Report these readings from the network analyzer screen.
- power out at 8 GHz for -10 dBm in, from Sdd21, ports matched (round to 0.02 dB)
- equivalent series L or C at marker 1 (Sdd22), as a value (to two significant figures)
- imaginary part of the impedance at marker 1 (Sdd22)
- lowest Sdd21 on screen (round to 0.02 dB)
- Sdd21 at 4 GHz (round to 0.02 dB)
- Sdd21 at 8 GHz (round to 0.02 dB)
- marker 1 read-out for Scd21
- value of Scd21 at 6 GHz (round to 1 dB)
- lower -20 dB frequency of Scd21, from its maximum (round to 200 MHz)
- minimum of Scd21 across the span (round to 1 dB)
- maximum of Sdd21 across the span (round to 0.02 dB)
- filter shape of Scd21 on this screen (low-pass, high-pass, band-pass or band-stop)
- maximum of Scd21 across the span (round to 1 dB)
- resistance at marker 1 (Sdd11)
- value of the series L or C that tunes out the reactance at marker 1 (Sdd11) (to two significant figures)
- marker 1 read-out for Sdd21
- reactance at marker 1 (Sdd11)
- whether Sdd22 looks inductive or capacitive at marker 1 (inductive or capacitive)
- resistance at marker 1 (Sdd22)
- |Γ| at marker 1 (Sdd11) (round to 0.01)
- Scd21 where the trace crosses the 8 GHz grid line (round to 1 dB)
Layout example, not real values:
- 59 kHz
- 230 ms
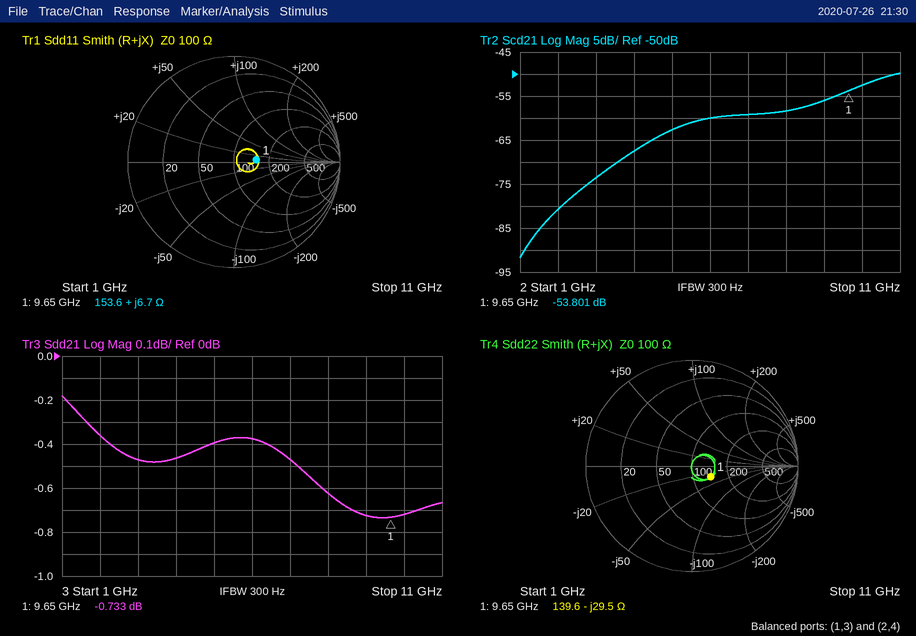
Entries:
- -10.62 dBm
- 560 fF
- -29.5 Ω
- -0.74 dB
- -0.46 dB
- -0.62 dB
- -53.801 dB
- -60 dB
- 3.6 GHz
- -92 dB
- -0.18 dB
- high-pass
- -50 dB
- 153.6 Ω
- 2.5 pF
- -0.733 dB
- +6.7 Ω
- capacitive
- 139.6 Ω
- 0.21
- -58 dB
